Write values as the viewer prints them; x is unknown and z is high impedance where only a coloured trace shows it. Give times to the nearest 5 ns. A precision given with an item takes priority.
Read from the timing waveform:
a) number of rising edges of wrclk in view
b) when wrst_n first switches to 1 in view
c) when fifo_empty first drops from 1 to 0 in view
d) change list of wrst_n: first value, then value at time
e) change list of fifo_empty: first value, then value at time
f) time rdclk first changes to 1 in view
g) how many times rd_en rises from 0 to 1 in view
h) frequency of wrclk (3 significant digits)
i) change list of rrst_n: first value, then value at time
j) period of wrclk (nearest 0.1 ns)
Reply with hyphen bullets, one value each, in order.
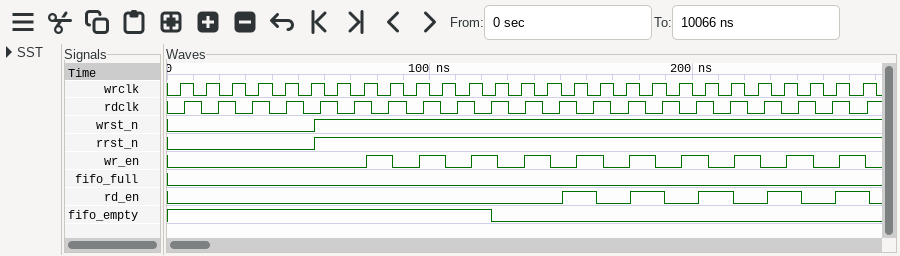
- 27
- 55 ns
- 125 ns
- 0, 1 at 55 ns
- 1, 0 at 125 ns
- 5 ns
- 5
- 100 MHz
- 0, 1 at 55 ns
- 10 ns
